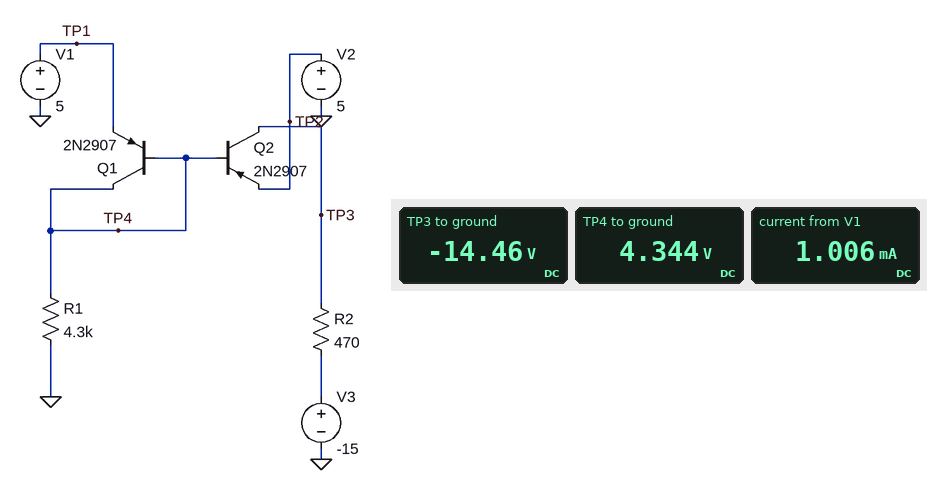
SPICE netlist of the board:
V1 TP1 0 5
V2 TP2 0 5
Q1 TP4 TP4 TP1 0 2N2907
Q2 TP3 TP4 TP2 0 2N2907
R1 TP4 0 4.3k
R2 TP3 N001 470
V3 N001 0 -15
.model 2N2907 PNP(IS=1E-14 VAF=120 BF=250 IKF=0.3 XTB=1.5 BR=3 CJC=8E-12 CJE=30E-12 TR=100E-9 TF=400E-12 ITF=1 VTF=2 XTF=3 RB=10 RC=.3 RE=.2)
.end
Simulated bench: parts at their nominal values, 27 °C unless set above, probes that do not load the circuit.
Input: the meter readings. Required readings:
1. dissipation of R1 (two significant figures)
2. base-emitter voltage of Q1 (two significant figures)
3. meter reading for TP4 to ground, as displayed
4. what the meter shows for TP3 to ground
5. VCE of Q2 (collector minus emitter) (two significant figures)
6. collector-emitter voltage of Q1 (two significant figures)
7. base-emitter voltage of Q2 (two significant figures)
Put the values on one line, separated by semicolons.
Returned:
4.4 mW; -660 mV; 4.344 V; -14.46 V; -19 V; -660 mV; -660 mV
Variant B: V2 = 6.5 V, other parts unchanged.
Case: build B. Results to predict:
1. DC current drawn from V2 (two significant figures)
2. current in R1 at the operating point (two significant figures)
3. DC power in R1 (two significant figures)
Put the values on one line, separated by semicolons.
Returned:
47 mA; 1.3 mA; 7.6 mW
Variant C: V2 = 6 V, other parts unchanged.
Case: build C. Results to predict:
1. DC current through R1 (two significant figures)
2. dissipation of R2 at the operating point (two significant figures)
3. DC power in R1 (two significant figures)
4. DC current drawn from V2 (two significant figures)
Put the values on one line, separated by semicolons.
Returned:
1.2 mA; 930 mW; 6.3 mW; 46 mA
